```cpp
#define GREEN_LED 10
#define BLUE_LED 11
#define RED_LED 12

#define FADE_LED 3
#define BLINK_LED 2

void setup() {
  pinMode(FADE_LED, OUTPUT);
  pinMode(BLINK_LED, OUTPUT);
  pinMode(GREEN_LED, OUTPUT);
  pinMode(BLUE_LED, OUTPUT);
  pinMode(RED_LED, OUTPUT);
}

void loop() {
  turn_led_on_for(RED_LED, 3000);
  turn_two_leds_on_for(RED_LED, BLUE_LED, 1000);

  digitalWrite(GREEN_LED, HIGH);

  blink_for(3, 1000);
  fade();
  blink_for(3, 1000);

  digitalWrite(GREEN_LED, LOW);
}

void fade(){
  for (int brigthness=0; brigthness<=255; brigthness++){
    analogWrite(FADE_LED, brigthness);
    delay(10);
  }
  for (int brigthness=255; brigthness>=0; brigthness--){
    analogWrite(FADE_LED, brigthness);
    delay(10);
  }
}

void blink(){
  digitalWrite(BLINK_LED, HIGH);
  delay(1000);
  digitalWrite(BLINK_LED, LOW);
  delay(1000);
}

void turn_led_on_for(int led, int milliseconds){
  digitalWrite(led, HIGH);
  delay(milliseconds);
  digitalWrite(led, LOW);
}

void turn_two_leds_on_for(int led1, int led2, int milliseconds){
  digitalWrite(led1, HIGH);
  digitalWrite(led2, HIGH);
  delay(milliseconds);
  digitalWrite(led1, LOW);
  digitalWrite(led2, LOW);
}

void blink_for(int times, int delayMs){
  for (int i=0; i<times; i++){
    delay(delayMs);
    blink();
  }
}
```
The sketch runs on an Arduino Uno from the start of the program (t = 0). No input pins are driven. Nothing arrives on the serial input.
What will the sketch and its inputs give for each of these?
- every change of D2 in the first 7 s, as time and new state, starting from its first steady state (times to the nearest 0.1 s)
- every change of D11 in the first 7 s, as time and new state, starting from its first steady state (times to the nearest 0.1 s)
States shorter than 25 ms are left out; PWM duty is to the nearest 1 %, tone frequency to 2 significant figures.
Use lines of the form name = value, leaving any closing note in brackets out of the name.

every change of D2 in the first 7 s, as time and new state, starting from its first steady state = 0 s low; 5 s high; 6 s low
every change of D11 in the first 7 s, as time and new state, starting from its first steady state = 0 s low; 3 s high; 4 s low
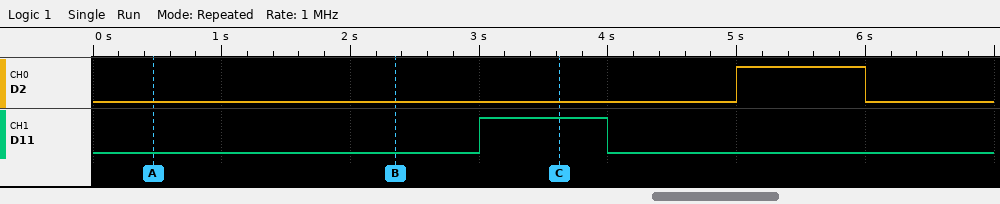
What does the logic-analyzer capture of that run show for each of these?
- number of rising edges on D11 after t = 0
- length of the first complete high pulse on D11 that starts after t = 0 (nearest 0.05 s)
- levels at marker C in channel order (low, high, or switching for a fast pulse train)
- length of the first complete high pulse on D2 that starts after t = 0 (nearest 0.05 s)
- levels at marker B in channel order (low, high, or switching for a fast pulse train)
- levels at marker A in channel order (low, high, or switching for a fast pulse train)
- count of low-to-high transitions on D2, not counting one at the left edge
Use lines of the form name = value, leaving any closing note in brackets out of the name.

number of rising edges on D11 after t = 0 = 1
length of the first complete high pulse on D11 that starts after t = 0 = 1.00 s
levels at marker C in channel order = D2 low, D11 high
length of the first complete high pulse on D2 that starts after t = 0 = 1.00 s
levels at marker B in channel order = D2 low, D11 low
levels at marker A in channel order = D2 low, D11 low
count of low-to-high transitions on D2, not counting one at the left edge = 1
